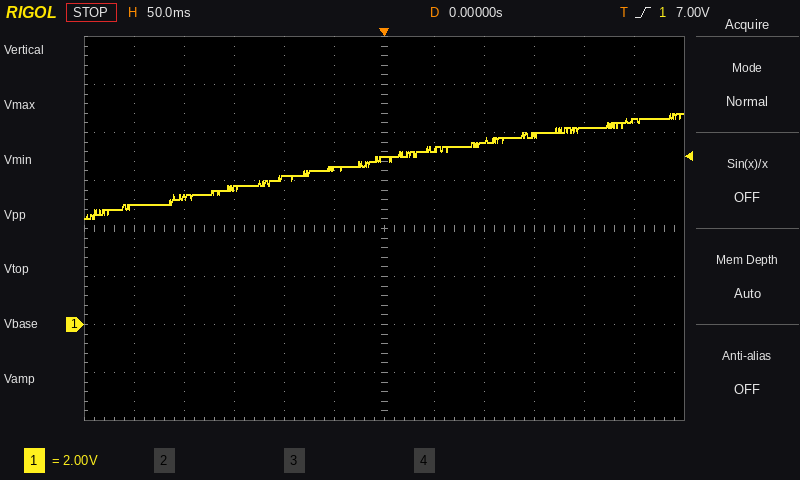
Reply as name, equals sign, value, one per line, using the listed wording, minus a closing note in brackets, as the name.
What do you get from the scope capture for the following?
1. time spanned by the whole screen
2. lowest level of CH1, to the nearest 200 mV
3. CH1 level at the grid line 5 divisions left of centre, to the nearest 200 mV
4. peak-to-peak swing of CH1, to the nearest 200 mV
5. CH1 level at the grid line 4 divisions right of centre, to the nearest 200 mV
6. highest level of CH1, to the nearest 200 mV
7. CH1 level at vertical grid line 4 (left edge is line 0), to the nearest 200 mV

time spanned by the whole screen = 600 ms
lowest level of CH1, to the nearest 200 mV = 4.4 V
CH1 level at the grid line 5 divisions left of centre, to the nearest 200 mV = 5.0 V
peak-to-peak swing of CH1, to the nearest 200 mV = 4.4 V
CH1 level at the grid line 4 divisions right of centre, to the nearest 200 mV = 8.2 V
highest level of CH1, to the nearest 200 mV = 8.8 V
CH1 level at vertical grid line 4 (left edge is line 0), to the nearest 200 mV = 6.2 V
